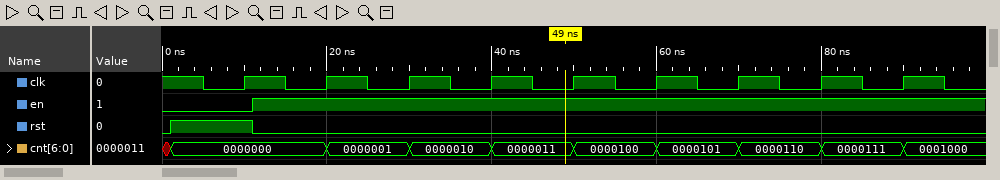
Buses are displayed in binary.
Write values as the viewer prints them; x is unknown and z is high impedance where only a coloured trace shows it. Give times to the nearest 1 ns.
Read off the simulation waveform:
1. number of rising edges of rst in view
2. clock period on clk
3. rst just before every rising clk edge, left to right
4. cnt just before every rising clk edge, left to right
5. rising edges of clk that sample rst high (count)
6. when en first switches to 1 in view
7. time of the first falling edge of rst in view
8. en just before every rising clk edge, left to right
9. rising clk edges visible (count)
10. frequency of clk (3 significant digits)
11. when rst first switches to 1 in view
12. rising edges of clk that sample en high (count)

1
10 ns
1 0 0 0 0 0 0 0 0
0000000, 0000000, 0000001, 0000010, 0000011, 0000100, 0000101, 0000110, 0000111
1
11 ns
11 ns
0 1 1 1 1 1 1 1 1
9
100 MHz
1 ns
8
